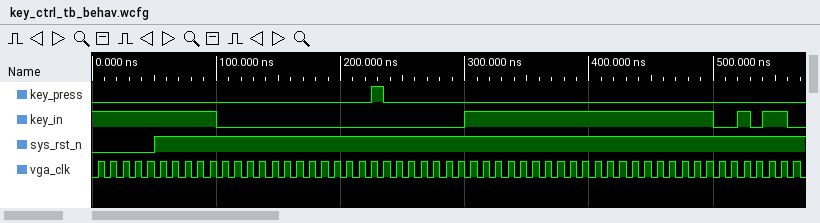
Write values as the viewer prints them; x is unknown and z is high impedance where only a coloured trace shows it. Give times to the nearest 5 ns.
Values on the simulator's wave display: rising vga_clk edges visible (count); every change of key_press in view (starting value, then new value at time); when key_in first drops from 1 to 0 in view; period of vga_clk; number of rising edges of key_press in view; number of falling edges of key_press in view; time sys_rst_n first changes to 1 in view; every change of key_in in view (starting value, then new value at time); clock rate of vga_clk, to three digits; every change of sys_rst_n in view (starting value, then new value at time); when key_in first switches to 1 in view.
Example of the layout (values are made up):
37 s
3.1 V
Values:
57
0, 1 at 225 ns, 0 at 235 ns
100 ns
10 ns
1
1
50 ns
1, 0 at 100 ns, 1 at 300 ns, 0 at 500 ns, 1 at 520 ns, 0 at 530 ns, 1 at 540 ns, 0 at 560 ns
100 MHz
0, 1 at 50 ns
300 ns
